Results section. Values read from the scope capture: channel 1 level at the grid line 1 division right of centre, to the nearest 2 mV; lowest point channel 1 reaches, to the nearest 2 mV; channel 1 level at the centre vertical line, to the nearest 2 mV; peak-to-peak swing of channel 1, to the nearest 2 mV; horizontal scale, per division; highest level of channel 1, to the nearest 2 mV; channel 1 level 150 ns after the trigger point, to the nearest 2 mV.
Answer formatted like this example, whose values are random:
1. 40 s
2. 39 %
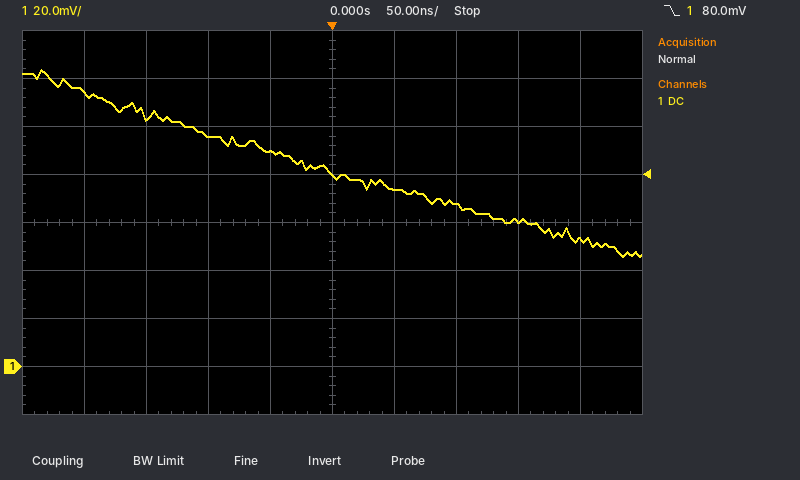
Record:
1. 74 mV
2. 46 mV
3. 80 mV
4. 78 mV
5. 50 ns
6. 124 mV
7. 60 mV
